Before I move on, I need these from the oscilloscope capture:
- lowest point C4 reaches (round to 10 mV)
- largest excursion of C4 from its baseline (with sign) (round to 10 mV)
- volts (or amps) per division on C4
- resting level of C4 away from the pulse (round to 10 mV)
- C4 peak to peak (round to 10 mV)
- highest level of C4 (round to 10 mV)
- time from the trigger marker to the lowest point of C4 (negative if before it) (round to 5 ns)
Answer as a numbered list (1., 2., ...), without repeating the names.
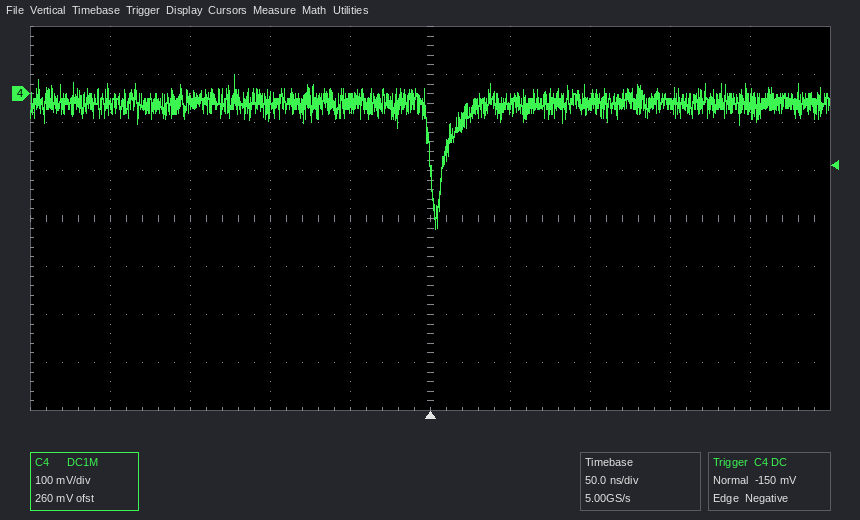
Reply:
1. -280 mV
2. -260 mV
3. 100 mV
4. -20 mV
5. 320 mV
6. 40 mV
7. +5 ns
